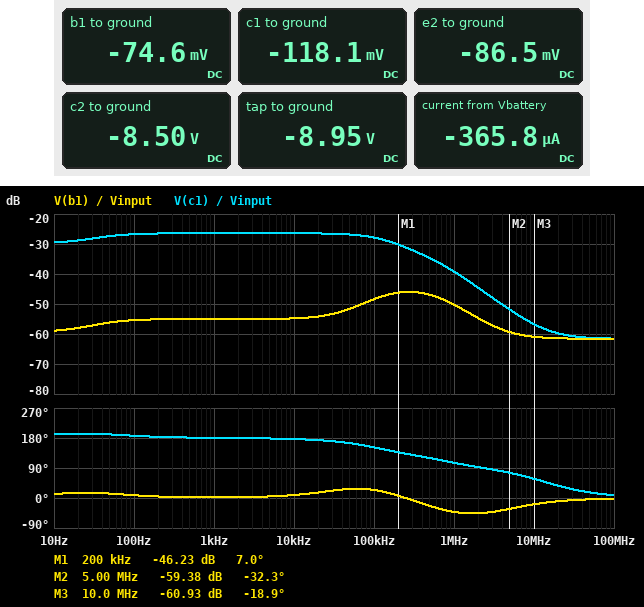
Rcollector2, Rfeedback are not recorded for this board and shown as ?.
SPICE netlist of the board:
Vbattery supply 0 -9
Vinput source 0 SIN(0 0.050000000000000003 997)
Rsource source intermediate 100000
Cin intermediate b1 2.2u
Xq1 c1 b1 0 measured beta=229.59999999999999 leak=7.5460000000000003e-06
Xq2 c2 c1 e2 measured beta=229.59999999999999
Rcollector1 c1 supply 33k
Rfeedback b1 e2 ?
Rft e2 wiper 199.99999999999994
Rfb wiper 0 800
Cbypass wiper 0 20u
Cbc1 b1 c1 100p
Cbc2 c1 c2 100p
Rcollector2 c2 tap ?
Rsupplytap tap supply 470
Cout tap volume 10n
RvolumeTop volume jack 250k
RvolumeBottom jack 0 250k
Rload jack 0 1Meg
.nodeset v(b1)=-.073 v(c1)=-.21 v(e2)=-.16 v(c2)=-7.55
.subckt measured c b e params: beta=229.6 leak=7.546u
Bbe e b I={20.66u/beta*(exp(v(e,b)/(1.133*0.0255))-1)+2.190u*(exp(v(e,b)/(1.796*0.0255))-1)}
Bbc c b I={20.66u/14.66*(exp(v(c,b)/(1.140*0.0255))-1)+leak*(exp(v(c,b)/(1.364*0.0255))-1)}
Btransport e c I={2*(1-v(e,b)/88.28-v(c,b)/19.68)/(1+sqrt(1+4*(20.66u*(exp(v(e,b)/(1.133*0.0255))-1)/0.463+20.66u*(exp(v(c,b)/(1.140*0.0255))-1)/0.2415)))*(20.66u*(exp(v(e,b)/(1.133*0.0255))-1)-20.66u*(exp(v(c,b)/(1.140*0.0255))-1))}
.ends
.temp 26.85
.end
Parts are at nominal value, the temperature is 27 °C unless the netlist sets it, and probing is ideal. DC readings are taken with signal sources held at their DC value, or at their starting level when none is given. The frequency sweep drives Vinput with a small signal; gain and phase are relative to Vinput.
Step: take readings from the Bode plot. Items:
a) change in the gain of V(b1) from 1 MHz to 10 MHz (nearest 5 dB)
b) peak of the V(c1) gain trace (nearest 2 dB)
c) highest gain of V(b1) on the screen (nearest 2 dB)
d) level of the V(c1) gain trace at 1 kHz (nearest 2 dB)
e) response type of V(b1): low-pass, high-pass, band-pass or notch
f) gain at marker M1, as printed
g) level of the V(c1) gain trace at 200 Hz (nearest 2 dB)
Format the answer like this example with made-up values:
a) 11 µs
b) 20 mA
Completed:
a) -10 dB
b) -26 dB
c) -46 dB
d) -26 dB
e) band-pass
f) -46.23 dB
g) -26 dB
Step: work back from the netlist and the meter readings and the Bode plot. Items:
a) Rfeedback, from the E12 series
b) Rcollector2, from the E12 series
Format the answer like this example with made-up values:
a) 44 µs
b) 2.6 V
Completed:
a) 3.3 kΩ
b) 4.7 kΩ
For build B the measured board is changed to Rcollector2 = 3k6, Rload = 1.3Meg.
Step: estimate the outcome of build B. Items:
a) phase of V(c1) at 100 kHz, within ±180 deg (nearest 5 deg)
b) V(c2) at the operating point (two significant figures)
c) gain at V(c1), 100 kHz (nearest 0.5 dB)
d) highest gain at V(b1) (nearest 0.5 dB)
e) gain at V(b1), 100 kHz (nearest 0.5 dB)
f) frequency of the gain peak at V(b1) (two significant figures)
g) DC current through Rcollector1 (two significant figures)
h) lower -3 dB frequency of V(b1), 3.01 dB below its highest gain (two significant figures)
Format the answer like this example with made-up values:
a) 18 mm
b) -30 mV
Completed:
a) 155 deg
b) -8.6 V
c) -27.5 dB
d) -46.5 dB
e) -49.5 dB
f) 310 kHz
g) 270 µA
h) 98 kHz
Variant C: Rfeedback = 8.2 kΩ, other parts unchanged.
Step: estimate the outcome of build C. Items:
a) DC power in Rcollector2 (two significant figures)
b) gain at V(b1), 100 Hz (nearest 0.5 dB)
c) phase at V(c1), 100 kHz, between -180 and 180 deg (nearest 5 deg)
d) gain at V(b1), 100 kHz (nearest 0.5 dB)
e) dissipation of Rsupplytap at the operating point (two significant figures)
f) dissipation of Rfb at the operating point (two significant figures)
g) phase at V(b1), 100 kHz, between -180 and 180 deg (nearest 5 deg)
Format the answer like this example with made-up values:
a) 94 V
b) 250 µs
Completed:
a) 52 µW
b) -52.0 dB
c) 140 deg
d) -44.5 dB
e) 5.2 µW
f) 7.5 µW
g) 15 deg
